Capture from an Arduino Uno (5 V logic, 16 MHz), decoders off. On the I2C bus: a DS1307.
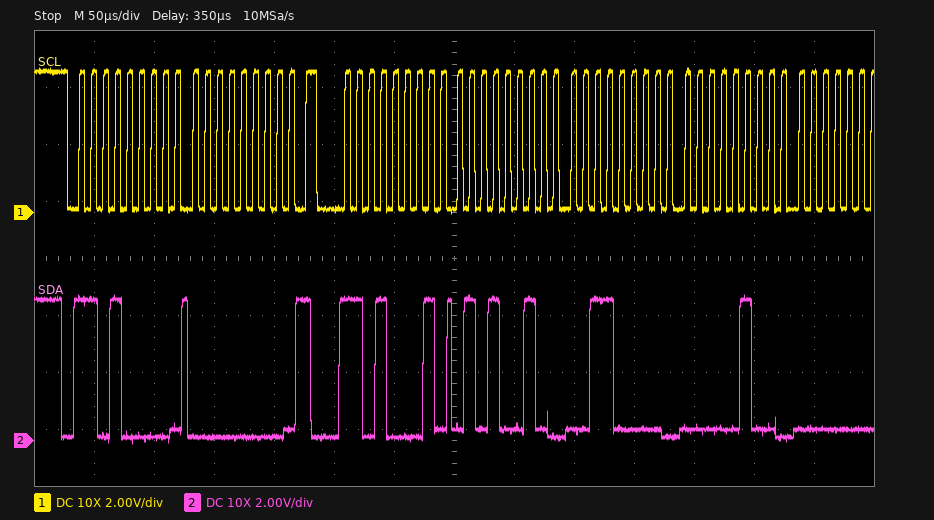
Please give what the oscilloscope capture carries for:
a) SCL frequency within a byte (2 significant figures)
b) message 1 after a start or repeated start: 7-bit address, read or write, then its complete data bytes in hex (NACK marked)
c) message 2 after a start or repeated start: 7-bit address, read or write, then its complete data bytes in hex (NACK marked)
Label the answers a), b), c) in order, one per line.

a) 100 kHz
b) 0x68 write: 00
c) 0x68 read: 52 30 04
